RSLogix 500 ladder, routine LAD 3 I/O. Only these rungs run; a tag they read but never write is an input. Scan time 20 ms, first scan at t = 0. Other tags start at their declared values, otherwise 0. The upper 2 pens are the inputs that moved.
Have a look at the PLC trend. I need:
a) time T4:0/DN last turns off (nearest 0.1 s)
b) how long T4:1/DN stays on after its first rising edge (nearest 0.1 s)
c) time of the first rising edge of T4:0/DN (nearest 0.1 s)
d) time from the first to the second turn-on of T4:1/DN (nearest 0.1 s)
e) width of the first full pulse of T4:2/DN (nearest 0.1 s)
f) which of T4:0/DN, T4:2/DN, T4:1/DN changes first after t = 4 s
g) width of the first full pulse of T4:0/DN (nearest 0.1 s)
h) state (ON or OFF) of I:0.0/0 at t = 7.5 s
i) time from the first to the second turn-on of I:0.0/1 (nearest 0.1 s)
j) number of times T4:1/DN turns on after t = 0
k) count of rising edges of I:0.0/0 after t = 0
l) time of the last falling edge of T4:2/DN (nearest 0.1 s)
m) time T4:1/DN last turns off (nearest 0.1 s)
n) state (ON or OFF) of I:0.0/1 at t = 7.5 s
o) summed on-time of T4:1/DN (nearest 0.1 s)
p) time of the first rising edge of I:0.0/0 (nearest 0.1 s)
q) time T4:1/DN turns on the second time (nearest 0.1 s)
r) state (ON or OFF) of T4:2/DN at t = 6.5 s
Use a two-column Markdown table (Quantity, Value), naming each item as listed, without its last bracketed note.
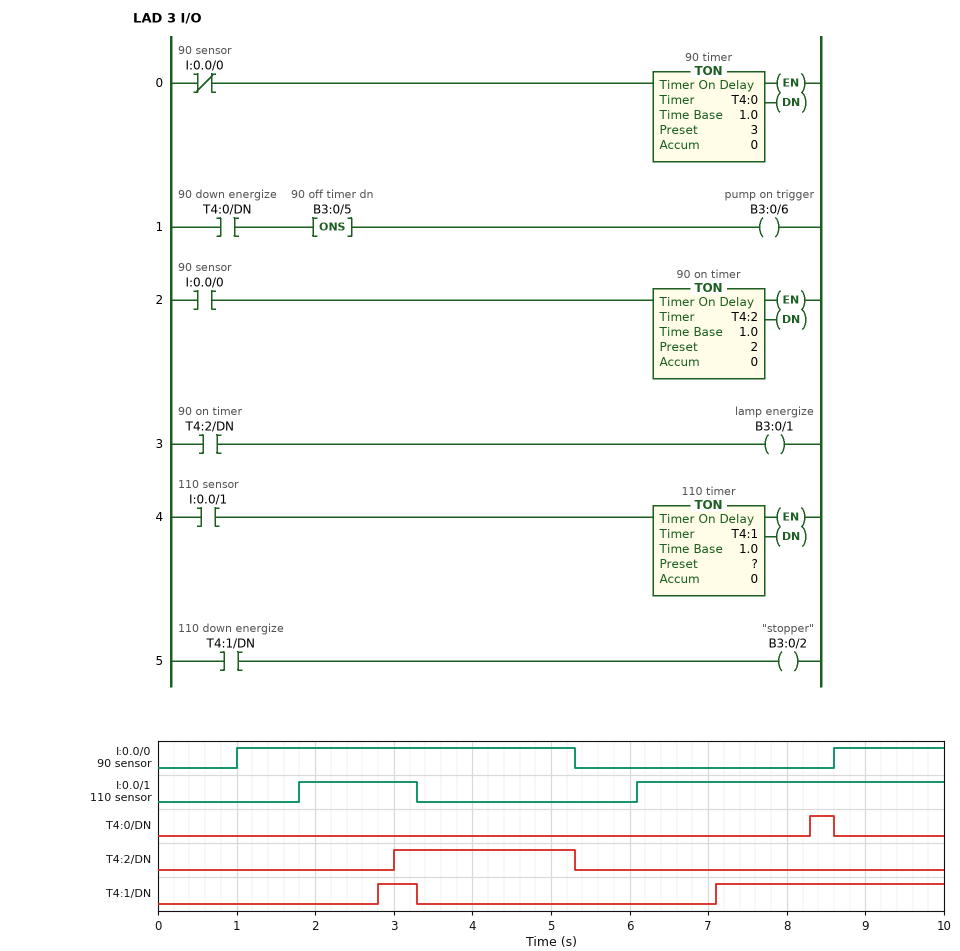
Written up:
| Quantity | Value |
|---|---|
| time T4:0/DN last turns off | 8.6 s |
| how long T4:1/DN stays on after its first rising edge | 0.5 s |
| time of the first rising edge of T4:0/DN | 8.3 s |
| time from the first to the second turn-on of T4:1/DN | 4.3 s |
| width of the first full pulse of T4:2/DN | 2.3 s |
| which of T4:0/DN, T4:2/DN, T4:1/DN changes first after t = 4 s | T4:2/DN |
| width of the first full pulse of T4:0/DN | 0.3 s |
| state (ON or OFF) of I:0.0/0 at t = 7.5 s | OFF |
| time from the first to the second turn-on of I:0.0/1 | 4.3 s |
| number of times T4:1/DN turns on after t = 0 | 2 |
| count of rising edges of I:0.0/0 after t = 0 | 2 |
| time of the last falling edge of T4:2/DN | 5.3 s |
| time T4:1/DN last turns off | 3.3 s |
| state (ON or OFF) of I:0.0/1 at t = 7.5 s | ON |
| summed on-time of T4:1/DN | 3.4 s |
| time of the first rising edge of I:0.0/0 | 1.0 s |
| time T4:1/DN turns on the second time | 7.1 s |
| state (ON or OFF) of T4:2/DN at t = 6.5 s | OFF |
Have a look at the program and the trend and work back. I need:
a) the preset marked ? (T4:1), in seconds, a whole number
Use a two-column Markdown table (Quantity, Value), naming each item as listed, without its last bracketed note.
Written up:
| Quantity | Value |
|---|---|
| the preset marked ? (T4:1), in seconds, a whole number | 1 s |
